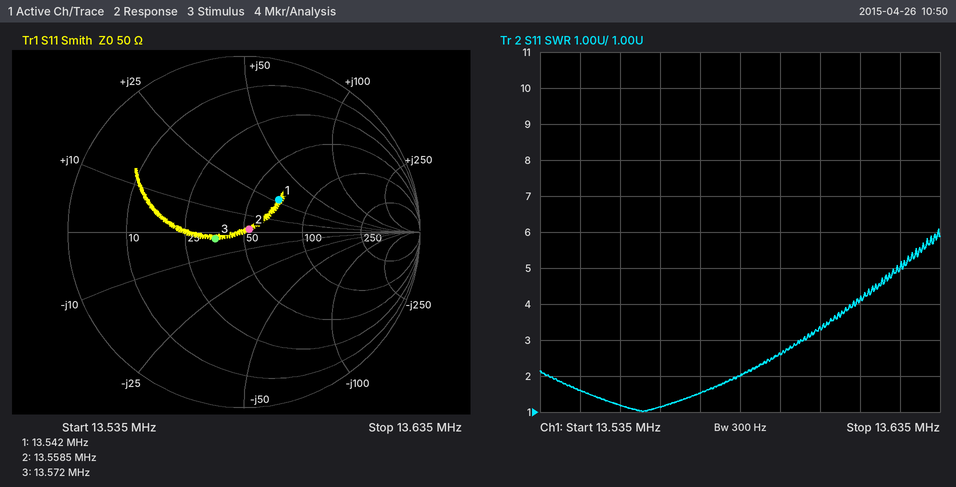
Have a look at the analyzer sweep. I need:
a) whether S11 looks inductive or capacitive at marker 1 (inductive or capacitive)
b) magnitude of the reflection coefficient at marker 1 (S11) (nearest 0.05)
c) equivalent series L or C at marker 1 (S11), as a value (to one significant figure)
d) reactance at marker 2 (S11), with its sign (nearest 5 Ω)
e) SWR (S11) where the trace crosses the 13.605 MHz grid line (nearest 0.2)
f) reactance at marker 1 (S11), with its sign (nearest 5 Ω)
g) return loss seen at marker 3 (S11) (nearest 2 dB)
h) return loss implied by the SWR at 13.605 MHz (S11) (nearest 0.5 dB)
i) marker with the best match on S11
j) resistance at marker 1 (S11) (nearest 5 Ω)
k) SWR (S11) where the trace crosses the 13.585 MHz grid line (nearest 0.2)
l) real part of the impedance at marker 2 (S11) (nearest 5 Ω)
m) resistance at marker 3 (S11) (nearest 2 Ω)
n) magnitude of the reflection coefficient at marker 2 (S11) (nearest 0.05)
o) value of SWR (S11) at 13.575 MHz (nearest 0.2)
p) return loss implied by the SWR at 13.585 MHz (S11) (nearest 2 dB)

inductive
0.25
300 nH
0 Ω
3.4
+25 Ω
16 dB
5.5 dB
marker 2
70 Ω
2.0
55 Ω
36 Ω
0.05
1.6
10 dB
